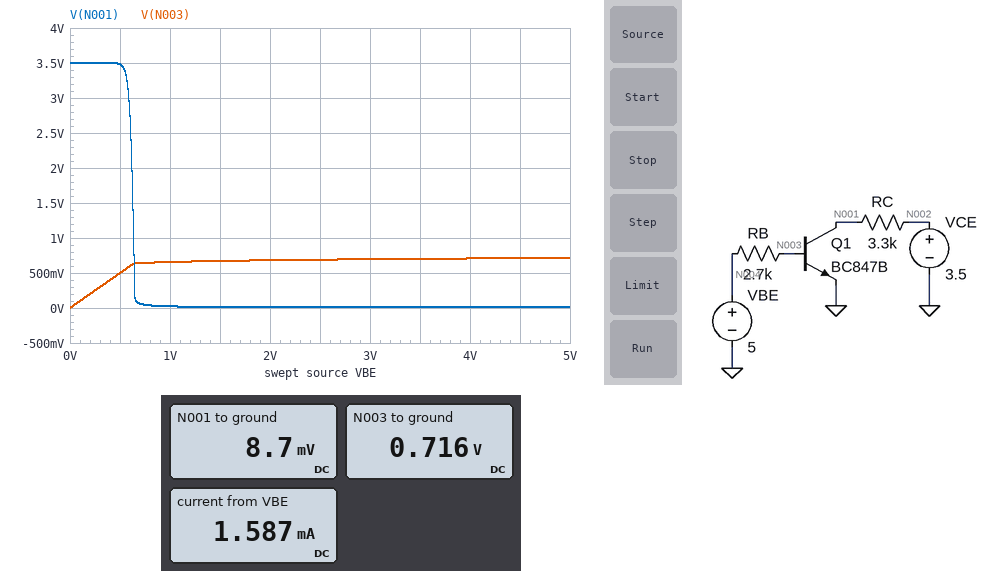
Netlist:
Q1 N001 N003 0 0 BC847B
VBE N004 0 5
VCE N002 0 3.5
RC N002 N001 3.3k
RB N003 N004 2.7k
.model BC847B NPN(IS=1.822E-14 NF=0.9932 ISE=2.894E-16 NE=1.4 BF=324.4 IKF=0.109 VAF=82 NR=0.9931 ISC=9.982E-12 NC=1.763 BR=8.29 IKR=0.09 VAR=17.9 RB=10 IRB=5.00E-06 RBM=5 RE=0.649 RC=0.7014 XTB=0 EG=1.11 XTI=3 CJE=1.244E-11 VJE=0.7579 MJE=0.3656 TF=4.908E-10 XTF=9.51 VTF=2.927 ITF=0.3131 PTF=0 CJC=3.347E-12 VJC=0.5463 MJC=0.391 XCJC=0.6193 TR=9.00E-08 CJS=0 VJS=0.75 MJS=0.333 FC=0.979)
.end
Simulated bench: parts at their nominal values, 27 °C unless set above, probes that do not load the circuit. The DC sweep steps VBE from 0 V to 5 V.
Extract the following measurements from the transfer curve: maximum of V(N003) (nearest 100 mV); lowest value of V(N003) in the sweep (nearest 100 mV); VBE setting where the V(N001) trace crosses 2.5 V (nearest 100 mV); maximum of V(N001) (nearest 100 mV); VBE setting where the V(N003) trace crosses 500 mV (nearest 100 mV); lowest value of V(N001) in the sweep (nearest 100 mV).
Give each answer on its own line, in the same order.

700 mV
0 V
600 mV
3.5 V
500 mV
0 V
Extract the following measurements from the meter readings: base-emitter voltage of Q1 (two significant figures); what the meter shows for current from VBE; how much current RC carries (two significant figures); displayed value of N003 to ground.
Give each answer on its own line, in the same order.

720 mV
1.587 mA
1.1 mA
0.716 V
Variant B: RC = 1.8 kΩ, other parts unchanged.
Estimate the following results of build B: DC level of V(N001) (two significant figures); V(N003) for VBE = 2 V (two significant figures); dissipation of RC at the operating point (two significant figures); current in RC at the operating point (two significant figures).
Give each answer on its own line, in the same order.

12 mV
690 mV
6.8 mW
1.9 mA
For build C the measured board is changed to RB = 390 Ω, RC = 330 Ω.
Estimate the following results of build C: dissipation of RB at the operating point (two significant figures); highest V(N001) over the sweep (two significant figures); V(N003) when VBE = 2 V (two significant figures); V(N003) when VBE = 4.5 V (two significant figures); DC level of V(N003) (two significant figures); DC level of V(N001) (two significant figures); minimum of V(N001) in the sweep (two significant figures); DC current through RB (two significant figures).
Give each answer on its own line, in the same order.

45 mW
3.5 V
760 mV
820 mV
830 mV
32 mV
31 mV
11 mA
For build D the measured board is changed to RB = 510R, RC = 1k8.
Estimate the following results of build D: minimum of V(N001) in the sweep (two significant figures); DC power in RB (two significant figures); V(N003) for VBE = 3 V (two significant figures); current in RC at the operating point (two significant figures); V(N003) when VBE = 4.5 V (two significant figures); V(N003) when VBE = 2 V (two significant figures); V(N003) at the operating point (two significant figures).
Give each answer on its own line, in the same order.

11 mV
35 mW
760 mV
1.9 mA
790 mV
730 mV
800 mV
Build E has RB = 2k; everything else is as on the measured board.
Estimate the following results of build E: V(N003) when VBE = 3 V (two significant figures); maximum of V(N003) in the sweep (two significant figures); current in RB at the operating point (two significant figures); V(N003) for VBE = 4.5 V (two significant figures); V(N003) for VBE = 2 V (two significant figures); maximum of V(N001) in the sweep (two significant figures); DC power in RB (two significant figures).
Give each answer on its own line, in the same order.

710 mV
730 mV
2.1 mA
720 mV
690 mV
3.5 V
9.1 mW
